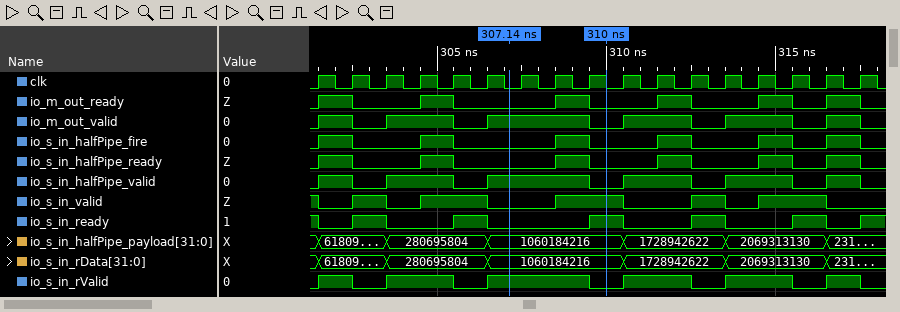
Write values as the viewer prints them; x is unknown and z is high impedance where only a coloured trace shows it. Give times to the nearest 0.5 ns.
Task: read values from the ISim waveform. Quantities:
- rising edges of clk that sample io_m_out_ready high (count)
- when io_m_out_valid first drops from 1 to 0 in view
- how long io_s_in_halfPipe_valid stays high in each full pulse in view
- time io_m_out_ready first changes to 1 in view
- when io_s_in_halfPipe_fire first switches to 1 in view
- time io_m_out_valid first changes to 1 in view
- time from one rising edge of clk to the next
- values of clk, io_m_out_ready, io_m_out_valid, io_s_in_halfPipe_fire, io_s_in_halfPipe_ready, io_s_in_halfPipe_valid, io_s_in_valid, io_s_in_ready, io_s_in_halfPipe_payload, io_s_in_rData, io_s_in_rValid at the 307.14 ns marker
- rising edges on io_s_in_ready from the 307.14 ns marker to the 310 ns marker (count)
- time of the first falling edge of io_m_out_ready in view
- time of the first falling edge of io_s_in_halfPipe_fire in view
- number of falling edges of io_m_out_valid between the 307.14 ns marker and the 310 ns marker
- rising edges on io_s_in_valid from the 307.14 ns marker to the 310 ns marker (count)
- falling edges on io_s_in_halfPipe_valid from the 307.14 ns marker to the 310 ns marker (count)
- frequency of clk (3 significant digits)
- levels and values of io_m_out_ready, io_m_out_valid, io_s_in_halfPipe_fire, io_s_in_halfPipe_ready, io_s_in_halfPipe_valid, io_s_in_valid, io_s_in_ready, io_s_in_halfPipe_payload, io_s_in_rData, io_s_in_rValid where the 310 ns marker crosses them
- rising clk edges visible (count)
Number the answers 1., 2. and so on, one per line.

1. 6
2. 302.5 ns
3. 1 ns, 2 ns, 3 ns, 2 ns, 2 ns, 1 ns
4. 301.5 ns
5. 301.5 ns
6. 301.5 ns
7. 1 ns
8. clk=0, io_m_out_ready=0, io_m_out_valid=1, io_s_in_halfPipe_fire=0, io_s_in_halfPipe_ready=0, io_s_in_halfPipe_valid=1, io_s_in_valid=0, io_s_in_ready=0, io_s_in_halfPipe_payload=1060184216, io_s_in_rData=1060184216, io_s_in_rValid=1
9. 1
10. 302.5 ns
11. 302.5 ns
12. 1
13. 1
14. 1
15. 1.00 GHz
16. io_m_out_ready=0, io_m_out_valid=0, io_s_in_halfPipe_fire=0, io_s_in_halfPipe_ready=0, io_s_in_halfPipe_valid=0, io_s_in_valid=1, io_s_in_ready=1, io_s_in_halfPipe_payload=1060184216, io_s_in_rData=1060184216, io_s_in_rValid=0
17. 17
